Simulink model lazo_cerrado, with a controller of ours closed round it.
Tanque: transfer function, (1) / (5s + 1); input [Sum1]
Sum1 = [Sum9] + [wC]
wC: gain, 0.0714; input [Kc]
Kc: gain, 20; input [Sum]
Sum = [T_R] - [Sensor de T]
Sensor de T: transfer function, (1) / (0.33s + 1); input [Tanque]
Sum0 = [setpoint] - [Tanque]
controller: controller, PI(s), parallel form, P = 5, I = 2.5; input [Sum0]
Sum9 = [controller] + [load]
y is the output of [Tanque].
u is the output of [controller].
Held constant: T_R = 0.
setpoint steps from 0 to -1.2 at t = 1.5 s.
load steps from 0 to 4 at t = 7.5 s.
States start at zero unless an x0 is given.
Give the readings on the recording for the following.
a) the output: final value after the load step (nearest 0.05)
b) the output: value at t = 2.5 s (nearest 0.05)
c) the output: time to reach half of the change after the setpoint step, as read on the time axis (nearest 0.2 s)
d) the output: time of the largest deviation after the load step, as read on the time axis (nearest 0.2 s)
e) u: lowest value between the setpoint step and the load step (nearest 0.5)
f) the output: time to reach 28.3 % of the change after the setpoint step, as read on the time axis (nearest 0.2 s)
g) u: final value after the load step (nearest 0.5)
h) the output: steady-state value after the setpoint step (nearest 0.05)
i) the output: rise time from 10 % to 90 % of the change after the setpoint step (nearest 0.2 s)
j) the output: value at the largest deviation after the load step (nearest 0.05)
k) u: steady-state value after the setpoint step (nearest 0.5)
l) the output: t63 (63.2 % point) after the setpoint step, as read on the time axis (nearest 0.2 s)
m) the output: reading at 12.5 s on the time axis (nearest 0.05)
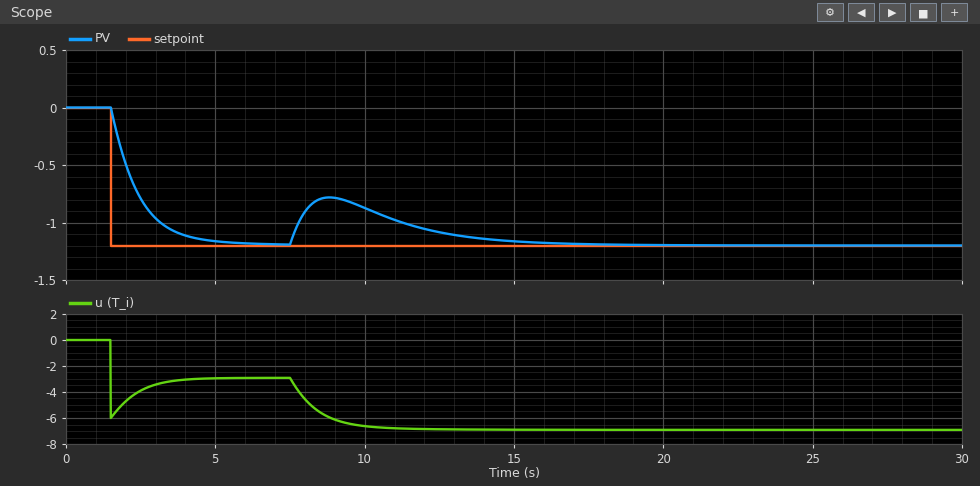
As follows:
-1.20
-0.80
2.2 s
8.8 s
-6.0
1.8 s
-7.0
-1.20
2.0 s
-0.80
-3.0
2.4 s
-1.10
